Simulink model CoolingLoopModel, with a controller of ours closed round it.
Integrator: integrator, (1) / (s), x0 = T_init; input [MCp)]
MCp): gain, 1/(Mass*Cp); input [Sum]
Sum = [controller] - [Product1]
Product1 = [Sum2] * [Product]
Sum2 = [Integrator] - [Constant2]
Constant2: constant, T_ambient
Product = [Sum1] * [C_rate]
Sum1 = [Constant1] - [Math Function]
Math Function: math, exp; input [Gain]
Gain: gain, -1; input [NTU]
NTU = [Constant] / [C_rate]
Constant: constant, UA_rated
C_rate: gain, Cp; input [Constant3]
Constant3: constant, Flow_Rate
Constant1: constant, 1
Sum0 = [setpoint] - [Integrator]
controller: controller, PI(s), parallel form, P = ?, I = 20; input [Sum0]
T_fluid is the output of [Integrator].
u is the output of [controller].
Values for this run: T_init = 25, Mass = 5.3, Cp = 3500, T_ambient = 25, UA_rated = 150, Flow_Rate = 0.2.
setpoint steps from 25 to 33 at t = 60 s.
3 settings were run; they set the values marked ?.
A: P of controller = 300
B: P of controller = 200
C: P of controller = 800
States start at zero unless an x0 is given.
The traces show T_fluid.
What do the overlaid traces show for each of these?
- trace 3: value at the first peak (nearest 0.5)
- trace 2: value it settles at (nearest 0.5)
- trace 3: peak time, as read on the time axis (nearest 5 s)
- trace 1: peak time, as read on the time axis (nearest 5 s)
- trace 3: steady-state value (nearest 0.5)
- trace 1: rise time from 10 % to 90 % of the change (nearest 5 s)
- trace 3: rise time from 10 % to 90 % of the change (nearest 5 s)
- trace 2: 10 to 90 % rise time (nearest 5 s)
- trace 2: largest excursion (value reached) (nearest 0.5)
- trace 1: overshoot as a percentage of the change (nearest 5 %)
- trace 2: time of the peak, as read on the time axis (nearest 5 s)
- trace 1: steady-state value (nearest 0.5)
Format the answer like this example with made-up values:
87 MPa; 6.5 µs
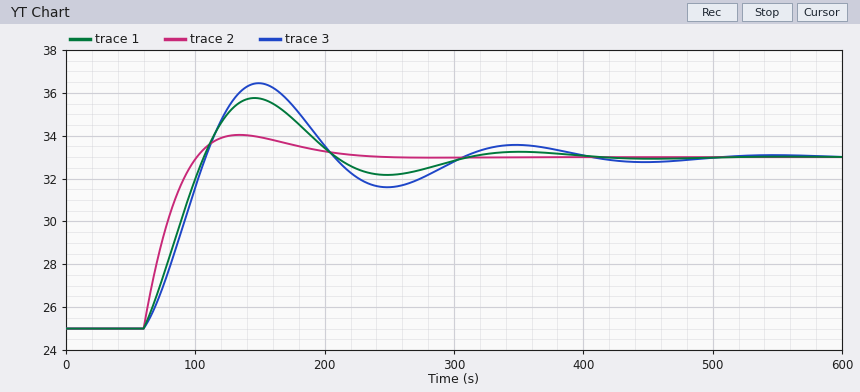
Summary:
36.5; 33.0; 150 s; 145 s; 33.0; 35 s; 35 s; 30 s; 34.0; 35 %; 135 s; 33.0
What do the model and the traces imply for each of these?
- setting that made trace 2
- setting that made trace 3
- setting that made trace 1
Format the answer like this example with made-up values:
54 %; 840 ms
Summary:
C; B; A
